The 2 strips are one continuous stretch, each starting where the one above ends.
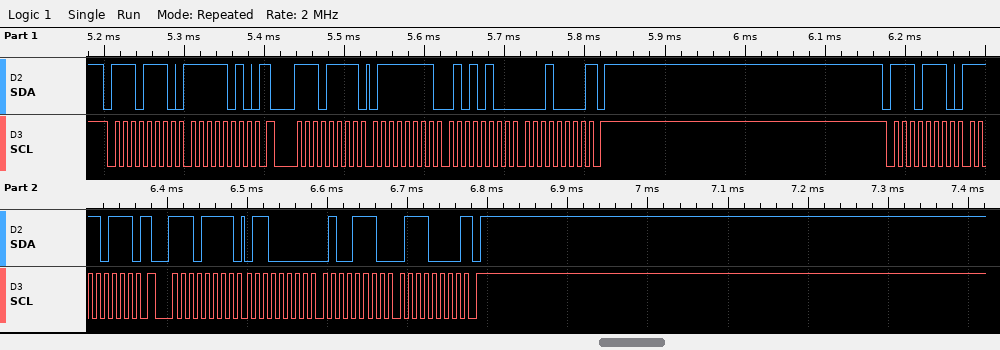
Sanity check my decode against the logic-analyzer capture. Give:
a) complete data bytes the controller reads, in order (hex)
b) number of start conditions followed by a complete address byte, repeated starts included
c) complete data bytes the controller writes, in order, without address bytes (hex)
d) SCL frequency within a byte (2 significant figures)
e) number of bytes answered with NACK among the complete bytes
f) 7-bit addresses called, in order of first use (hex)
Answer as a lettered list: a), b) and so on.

a) 7F 54 10 60 4E 70
b) 4
c) FA F7
d) 100 kHz
e) 2
f) 0x77
